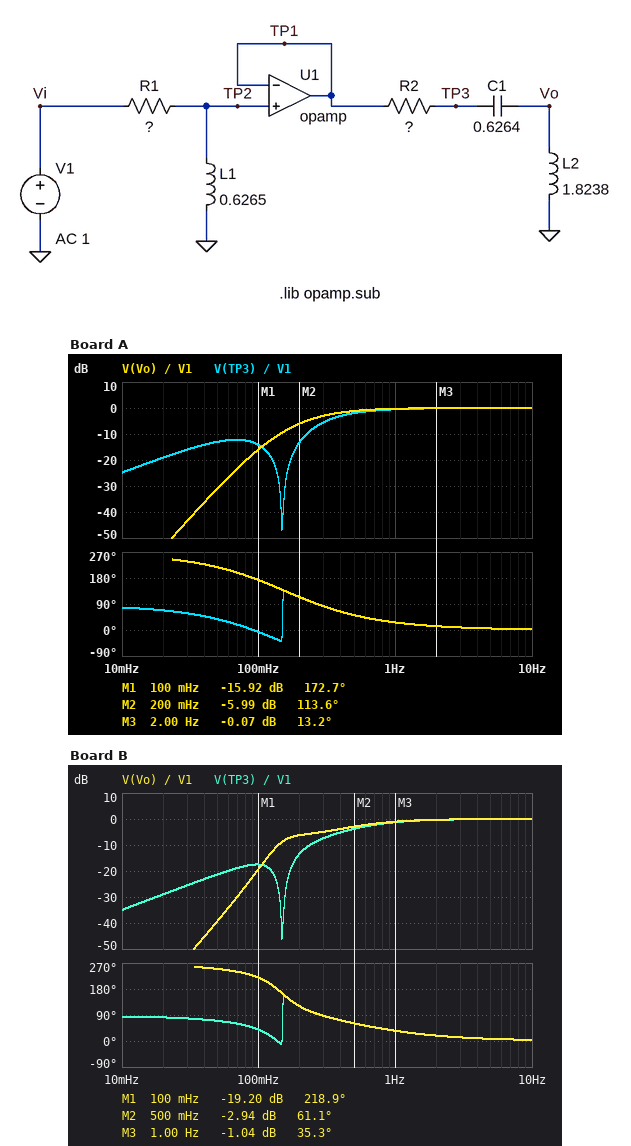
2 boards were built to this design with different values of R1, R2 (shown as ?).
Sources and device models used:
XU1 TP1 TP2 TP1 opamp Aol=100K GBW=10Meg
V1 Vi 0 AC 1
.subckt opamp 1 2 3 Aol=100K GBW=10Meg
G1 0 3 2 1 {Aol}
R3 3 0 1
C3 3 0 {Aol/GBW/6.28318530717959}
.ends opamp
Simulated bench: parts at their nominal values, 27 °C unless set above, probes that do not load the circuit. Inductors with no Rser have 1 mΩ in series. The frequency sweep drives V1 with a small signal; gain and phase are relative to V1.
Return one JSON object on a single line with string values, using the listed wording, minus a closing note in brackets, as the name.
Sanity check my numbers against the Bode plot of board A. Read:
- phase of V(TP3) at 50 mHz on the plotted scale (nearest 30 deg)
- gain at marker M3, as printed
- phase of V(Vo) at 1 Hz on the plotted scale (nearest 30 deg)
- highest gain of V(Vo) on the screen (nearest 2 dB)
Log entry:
{"phase of V(TP3) at 50 mHz on the plotted scale": "30 deg", "gain at marker M3, as printed": "-0.07 dB", "phase of V(Vo) at 1 Hz on the plotted scale": "30 deg", "highest gain of V(Vo) on the screen": "0 dB"}
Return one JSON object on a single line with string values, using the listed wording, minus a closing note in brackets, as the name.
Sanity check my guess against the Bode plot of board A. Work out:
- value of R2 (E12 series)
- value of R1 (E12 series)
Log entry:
{"value of R2": "3.3 Ω", "value of R1": "0.68 Ω"}
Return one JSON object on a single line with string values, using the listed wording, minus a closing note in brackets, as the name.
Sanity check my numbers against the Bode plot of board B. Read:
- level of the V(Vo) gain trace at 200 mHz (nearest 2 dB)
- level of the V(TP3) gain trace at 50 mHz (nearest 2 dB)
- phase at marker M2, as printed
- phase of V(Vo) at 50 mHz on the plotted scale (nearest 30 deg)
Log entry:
{"level of the V(Vo) gain trace at 200 mHz": "-6 dB", "level of the V(TP3) gain trace at 50 mHz": "-22 dB", "phase at marker M2, as printed": "61.1 deg", "phase of V(Vo) at 50 mHz on the plotted scale": "240 deg"}
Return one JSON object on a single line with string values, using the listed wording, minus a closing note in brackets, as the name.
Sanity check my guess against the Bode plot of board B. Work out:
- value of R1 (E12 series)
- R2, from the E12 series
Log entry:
{"value of R1": "2.2 Ω", "R2, from the E12 series": "1.2 Ω"}
